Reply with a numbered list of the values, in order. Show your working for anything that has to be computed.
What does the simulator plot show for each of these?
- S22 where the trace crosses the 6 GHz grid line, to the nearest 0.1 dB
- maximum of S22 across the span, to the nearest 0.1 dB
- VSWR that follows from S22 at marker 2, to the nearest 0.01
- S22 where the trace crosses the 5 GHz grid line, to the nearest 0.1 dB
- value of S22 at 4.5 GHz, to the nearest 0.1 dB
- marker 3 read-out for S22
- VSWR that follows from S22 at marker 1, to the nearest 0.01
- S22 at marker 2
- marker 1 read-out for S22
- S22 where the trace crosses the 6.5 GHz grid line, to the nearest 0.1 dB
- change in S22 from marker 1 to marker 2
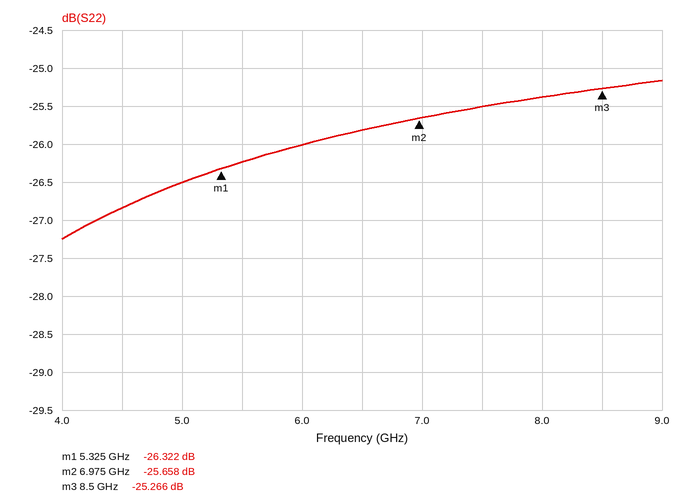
1. -26.0 dB
2. -25.2 dB
3. (1 + 0.0521)/(1 − 0.0521) ≈ 1.11
4. -26.5 dB
5. -26.8 dB
6. -25.266 dB
7. (1 + 0.0483)/(1 − 0.0483) ≈ 1.10
8. -25.658 dB
9. -26.322 dB
10. -25.8 dB
11. -25.658 − (-26.322) = 0.664 dB
